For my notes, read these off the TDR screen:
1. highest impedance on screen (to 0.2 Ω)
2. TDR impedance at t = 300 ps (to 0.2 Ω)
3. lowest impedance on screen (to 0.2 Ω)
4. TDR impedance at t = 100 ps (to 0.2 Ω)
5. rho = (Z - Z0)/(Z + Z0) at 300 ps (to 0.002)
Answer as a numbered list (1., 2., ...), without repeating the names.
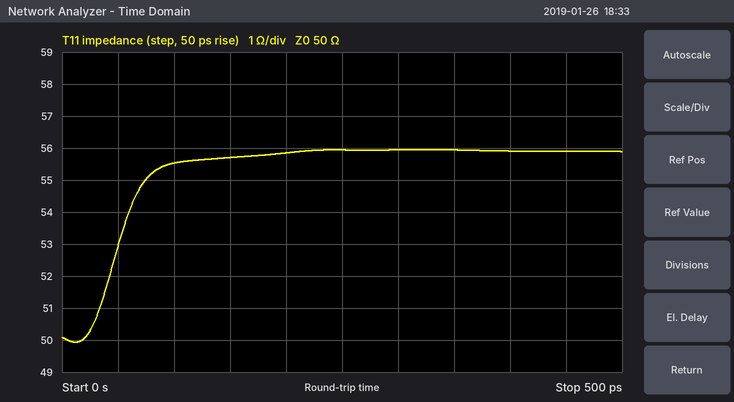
1. 56.0 Ω
2. 56.0 Ω
3. 50.0 Ω
4. 55.6 Ω
5. +0.056
